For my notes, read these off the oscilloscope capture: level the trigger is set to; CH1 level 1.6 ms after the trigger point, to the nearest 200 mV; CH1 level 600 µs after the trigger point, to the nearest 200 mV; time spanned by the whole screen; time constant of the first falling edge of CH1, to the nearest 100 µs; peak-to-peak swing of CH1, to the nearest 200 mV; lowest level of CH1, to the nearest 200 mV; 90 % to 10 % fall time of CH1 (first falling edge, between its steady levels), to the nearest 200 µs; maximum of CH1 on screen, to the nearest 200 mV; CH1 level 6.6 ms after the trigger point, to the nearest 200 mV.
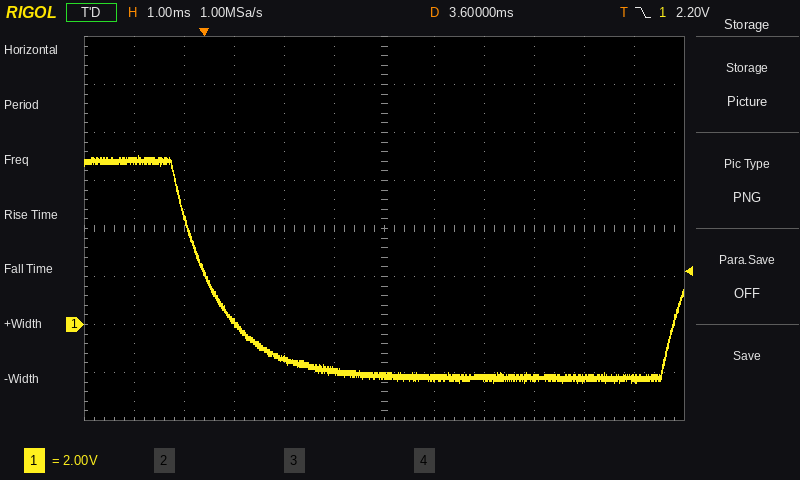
2.20 V
-1.4 V
200 mV
12 ms
900 µs
9.4 V
-2.4 V
2.0 ms
7.0 V
-2.2 V
